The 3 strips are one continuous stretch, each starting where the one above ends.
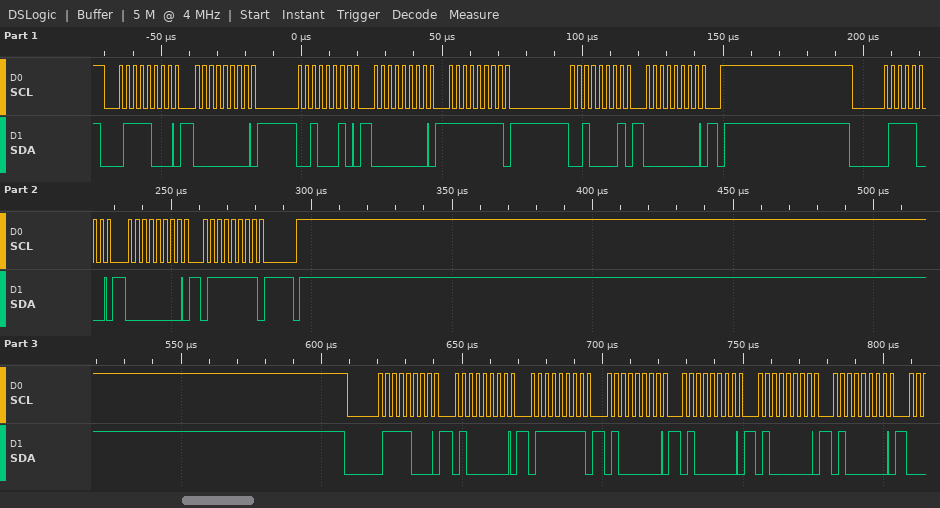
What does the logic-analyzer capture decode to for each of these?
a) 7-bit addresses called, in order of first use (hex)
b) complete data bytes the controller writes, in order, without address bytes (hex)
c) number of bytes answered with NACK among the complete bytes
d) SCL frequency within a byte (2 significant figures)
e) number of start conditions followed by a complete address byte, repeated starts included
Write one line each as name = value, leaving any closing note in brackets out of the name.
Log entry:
7-bit addresses called, in order of first use = 0x3C
complete data bytes the controller writes, in order, without address bytes = 00 22 00 FF 21 00 00 7F 40 7F 40 40 40 40
number of bytes answered with NACK among the complete bytes = 0
SCL frequency within a byte = 400 kHz
number of start conditions followed by a complete address byte, repeated starts included = 3
